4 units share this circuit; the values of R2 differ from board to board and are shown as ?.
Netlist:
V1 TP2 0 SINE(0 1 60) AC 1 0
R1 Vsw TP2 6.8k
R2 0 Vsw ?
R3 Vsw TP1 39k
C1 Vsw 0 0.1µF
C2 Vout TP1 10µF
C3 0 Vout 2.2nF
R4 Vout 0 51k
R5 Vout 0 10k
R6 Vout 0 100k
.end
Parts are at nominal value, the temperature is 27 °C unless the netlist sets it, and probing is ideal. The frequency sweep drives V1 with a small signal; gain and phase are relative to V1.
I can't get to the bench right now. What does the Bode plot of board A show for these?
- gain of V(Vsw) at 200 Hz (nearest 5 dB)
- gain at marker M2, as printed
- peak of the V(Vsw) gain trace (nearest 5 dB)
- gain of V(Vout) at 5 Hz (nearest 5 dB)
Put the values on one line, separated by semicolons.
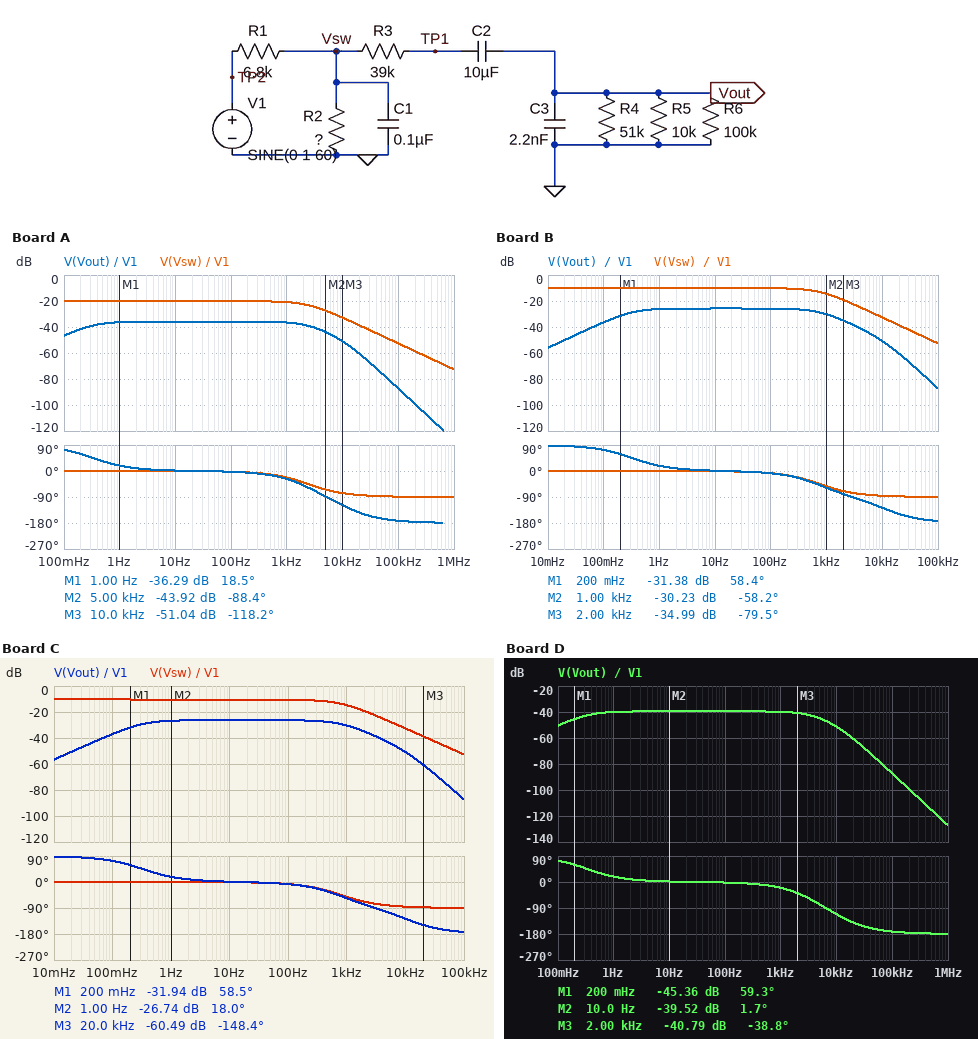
-20 dB; -43.92 dB; -20 dB; -35 dB
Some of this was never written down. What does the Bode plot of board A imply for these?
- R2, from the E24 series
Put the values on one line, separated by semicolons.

750 Ω
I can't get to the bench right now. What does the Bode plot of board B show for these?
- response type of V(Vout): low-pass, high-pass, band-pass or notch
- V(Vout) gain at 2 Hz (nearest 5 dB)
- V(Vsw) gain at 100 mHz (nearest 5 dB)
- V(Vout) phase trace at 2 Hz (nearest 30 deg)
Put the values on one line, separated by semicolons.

band-pass; -25 dB; -10 dB; 0 deg
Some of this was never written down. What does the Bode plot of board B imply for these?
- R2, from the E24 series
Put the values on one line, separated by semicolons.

3.3 kΩ
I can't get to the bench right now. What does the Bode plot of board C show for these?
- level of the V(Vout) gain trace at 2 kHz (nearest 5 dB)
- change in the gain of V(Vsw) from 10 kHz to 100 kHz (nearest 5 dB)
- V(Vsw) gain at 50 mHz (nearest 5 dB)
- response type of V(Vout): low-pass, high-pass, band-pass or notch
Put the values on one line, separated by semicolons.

-35 dB; -20 dB; -10 dB; band-pass
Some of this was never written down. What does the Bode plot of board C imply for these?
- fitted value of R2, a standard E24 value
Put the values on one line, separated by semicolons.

3 kΩ
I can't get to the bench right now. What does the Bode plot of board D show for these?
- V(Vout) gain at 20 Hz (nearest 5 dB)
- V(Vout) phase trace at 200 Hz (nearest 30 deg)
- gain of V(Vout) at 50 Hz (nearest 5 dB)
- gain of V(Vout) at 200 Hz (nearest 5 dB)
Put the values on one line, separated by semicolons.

-40 dB; 0 deg; -40 dB; -40 dB
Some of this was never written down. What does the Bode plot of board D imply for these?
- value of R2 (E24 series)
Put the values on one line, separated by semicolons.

470 Ω
